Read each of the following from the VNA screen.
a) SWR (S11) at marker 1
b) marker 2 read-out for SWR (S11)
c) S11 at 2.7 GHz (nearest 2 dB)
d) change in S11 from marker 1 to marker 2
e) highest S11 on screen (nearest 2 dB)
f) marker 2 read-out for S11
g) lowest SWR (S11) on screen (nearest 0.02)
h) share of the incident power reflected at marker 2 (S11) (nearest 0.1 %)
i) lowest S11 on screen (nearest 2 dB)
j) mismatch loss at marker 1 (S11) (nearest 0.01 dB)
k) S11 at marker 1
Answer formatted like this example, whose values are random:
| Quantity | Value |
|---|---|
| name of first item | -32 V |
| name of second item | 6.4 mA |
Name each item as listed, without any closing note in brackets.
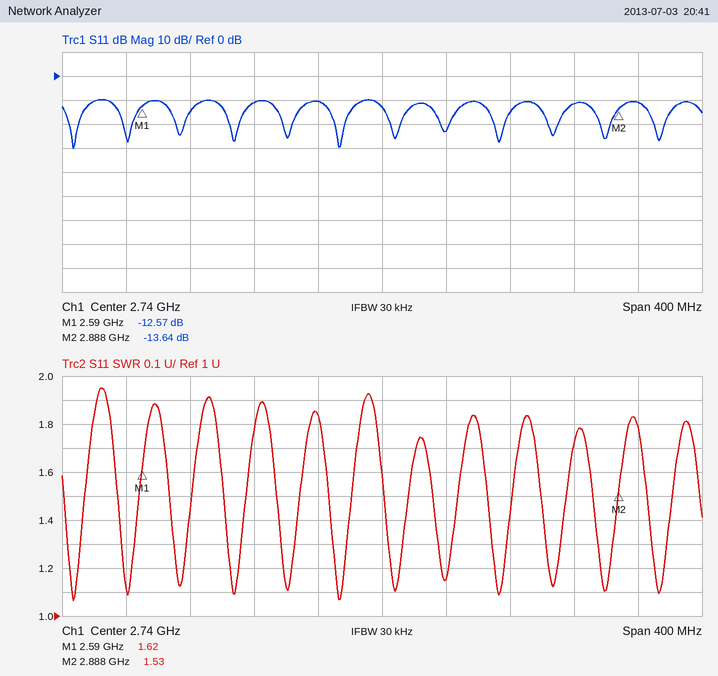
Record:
| Quantity | Value |
|---|---|
| SWR (S11) at marker 1 | 1.62 |
| marker 2 read-out for SWR | 1.53 |
| S11 at 2.7 GHz | -10 dB |
| change in S11 from marker 1 to marker 2 | -1.07 dB |
| highest S11 on screen | -10 dB |
| marker 2 read-out for S11 | -13.64 dB |
| lowest SWR (S11) on screen | 1.06 |
| share of the incident power reflected at marker 2 (S11) | 4.3 % |
| lowest S11 on screen | -30 dB |
| mismatch loss at marker 1 (S11) | 0.25 dB |
| S11 at marker 1 | -12.57 dB |
